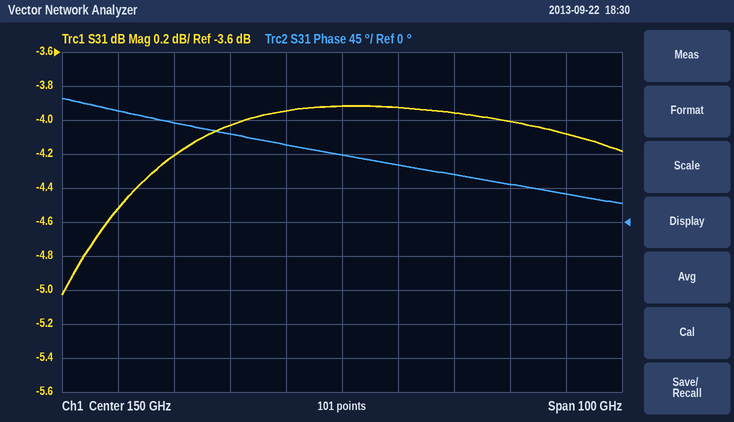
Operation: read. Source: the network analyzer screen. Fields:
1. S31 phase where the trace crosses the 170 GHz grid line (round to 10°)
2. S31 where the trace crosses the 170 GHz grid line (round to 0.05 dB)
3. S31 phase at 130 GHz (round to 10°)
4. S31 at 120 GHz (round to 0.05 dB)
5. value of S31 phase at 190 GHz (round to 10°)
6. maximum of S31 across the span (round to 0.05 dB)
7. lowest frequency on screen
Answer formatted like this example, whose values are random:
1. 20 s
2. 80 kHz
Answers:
1. 60°
2. -3.95 dB
3. 120°
4. -4.20 dB
5. 40°
6. -3.90 dB
7. 100 GHz
